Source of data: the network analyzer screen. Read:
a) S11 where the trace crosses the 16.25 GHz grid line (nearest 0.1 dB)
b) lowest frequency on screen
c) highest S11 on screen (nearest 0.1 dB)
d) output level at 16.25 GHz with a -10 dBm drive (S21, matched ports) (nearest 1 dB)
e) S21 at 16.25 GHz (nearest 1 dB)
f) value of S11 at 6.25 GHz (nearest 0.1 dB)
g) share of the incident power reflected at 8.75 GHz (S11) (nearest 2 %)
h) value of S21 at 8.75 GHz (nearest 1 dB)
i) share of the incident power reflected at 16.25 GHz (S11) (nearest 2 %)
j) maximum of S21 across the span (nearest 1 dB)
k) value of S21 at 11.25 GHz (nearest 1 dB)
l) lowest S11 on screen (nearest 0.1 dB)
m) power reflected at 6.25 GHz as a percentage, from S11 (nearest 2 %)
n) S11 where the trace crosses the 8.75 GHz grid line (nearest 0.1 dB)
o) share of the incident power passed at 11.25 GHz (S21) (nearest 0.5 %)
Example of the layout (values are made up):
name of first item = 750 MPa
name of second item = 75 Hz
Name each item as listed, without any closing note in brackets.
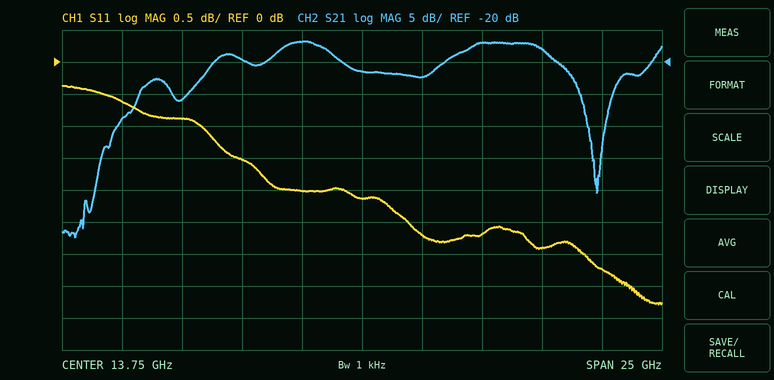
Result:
S11 where the trace crosses the 16.25 GHz grid line = -2.7 dB
lowest frequency on screen = 1.25 GHz
highest S11 on screen = -0.4 dB
output level at 16.25 GHz with a -10 dBm drive (S21, matched ports) = -32 dBm
S21 at 16.25 GHz = -22 dB
value of S11 at 6.25 GHz = -0.9 dB
share of the incident power reflected at 8.75 GHz (S11) = 70 %
value of S21 at 8.75 GHz = -20 dB
share of the incident power reflected at 16.25 GHz (S11) = 54 %
maximum of S21 across the span = -17 dB
value of S21 at 11.25 GHz = -17 dB
lowest S11 on screen = -3.8 dB
power reflected at 6.25 GHz as a percentage, from S11 = 82 %
S11 where the trace crosses the 8.75 GHz grid line = -1.5 dB
share of the incident power passed at 11.25 GHz (S21) = 2.0 %
